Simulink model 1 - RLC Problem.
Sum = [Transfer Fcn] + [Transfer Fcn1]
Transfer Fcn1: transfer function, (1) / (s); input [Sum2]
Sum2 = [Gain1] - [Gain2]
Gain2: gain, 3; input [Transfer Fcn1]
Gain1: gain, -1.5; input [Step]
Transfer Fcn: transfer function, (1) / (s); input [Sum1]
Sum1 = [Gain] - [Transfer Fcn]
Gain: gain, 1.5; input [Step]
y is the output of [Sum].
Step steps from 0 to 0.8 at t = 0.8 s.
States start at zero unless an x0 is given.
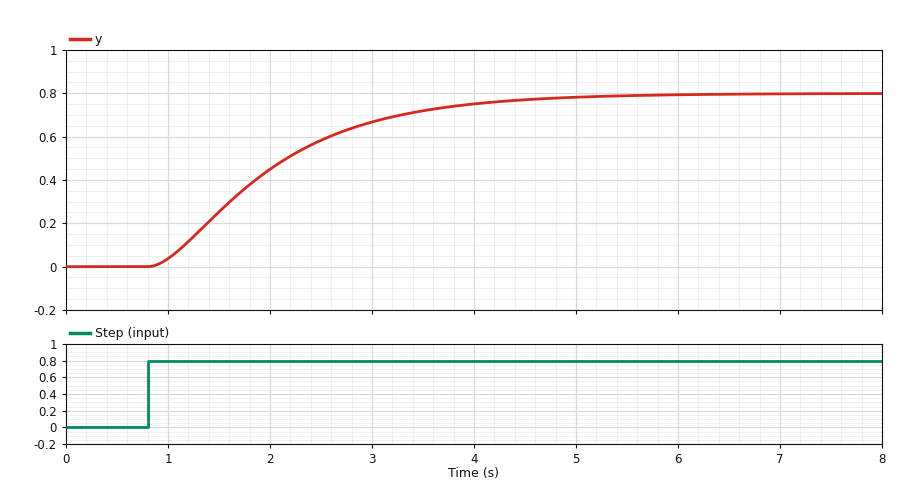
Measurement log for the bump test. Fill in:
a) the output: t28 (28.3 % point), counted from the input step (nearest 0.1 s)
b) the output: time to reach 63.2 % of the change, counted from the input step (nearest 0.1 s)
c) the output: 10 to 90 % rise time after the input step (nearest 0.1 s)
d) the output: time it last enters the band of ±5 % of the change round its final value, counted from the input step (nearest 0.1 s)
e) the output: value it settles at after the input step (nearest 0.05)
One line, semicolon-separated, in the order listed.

0.6 s; 1.4 s; 2.4 s; 3.4 s; 0.80
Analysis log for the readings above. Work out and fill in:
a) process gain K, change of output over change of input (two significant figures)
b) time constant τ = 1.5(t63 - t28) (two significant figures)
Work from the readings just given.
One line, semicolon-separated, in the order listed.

1.0; 1.2 s
